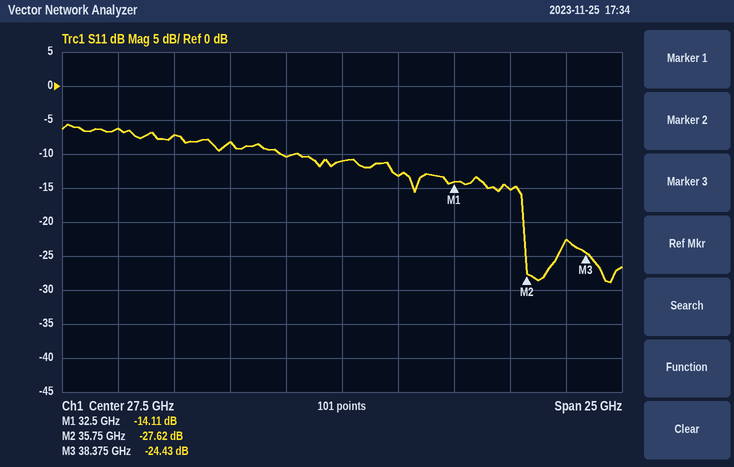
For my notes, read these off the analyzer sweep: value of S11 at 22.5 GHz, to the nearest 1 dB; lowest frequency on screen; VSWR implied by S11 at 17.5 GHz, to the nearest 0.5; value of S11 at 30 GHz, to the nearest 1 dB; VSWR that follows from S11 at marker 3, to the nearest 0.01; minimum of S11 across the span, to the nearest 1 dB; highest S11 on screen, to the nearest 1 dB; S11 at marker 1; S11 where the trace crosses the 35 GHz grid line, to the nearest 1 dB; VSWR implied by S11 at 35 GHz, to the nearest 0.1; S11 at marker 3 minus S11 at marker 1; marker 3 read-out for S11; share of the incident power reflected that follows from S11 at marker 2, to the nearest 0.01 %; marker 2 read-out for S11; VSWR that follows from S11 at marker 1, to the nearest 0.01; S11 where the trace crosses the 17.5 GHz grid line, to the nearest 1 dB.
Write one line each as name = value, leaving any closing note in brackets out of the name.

value of S11 at 22.5 GHz, to the nearest 1 dB = -8 dB
lowest frequency on screen = 15 GHz
VSWR implied by S11 at 17.5 GHz, to the nearest 0.5 = 3.0
value of S11 at 30 GHz, to the nearest 1 dB = -13 dB
VSWR that follows from S11 at marker 3, to the nearest 0.01 = 1.13
minimum of S11 across the span, to the nearest 1 dB = -29 dB
highest S11 on screen, to the nearest 1 dB = -6 dB
S11 at marker 1 = -14.11 dB
S11 where the trace crosses the 35 GHz grid line, to the nearest 1 dB = -15 dB
VSWR implied by S11 at 35 GHz, to the nearest 0.1 = 1.4
S11 at marker 3 minus S11 at marker 1 = -10.32 dB
marker 3 read-out for S11 = -24.43 dB
share of the incident power reflected that follows from S11 at marker 2, to the nearest 0.01 % = 0.17 %
marker 2 read-out for S11 = -27.62 dB
VSWR that follows from S11 at marker 1, to the nearest 0.01 = 1.49
S11 where the trace crosses the 17.5 GHz grid line, to the nearest 1 dB = -6 dB
